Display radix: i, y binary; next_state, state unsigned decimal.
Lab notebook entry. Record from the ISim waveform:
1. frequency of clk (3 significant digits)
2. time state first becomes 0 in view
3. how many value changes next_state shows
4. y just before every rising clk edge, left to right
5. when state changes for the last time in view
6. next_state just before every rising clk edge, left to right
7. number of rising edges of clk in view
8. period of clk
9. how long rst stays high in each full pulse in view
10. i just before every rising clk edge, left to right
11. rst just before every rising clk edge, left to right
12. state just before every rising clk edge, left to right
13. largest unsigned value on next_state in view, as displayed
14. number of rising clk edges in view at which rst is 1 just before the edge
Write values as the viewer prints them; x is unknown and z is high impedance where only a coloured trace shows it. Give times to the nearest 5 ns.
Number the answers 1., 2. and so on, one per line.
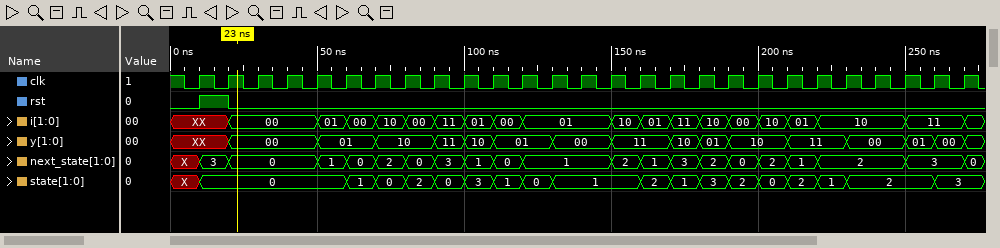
1. 100 MHz
2. 10 ns
3. 20
4. XX, XX, 00, 00, 00, 01, 01, 10, 10, 11, 10, 01, 01, 00, 00, 11, 11, 10, 01, 10, 10, 11, 11, 00, 00, 01, 00
5. 260 ns
6. X, 3, 0, 0, 0, 1, 0, 2, 0, 3, 1, 0, 1, 1, 1, 2, 1, 3, 2, 0, 2, 1, 2, 2, 2, 3, 3
7. 27
8. 10 ns
9. 10 ns
10. XX, XX, 00, 00, 00, 01, 00, 10, 00, 11, 01, 00, 01, 01, 01, 10, 01, 11, 10, 00, 10, 01, 10, 10, 10, 11, 11
11. 0 1 0 0 0 0 0 0 0 0 0 0 0 0 0 0 0 0 0 0 0 0 0 0 0 0 0
12. X, 0, 0, 0, 0, 0, 1, 0, 2, 0, 3, 1, 0, 1, 1, 1, 2, 1, 3, 2, 0, 2, 1, 2, 2, 2, 3
13. 3
14. 1
